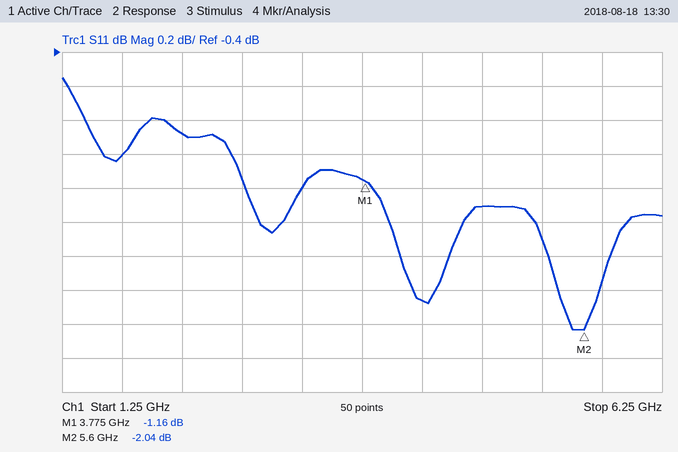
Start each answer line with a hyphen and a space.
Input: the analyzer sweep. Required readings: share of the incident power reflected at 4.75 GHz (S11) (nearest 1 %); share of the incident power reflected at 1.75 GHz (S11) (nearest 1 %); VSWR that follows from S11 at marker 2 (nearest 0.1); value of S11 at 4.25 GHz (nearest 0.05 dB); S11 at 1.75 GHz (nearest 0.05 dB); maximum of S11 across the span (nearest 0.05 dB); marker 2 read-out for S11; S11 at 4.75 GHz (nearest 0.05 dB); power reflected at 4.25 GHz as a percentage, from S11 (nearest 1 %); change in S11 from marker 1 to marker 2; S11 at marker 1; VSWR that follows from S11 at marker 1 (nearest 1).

- 74 %
- 79 %
- 8.6
- -1.85 dB
- -1.00 dB
- -0.55 dB
- -2.04 dB
- -1.30 dB
- 65 %
- -0.88 dB
- -1.16 dB
- 15
